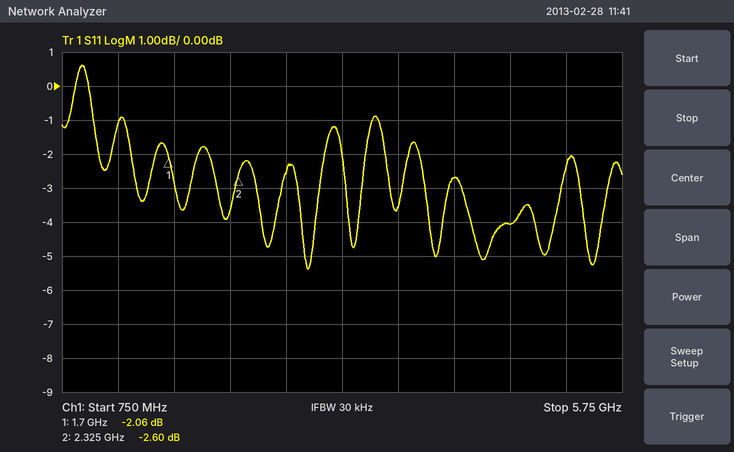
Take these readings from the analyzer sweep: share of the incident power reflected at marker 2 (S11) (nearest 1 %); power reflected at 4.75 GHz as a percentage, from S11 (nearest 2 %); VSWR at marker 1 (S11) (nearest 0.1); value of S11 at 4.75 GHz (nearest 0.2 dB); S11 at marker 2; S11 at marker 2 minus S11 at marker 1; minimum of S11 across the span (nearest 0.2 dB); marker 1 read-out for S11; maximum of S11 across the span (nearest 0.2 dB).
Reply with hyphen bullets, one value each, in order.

- 55 %
- 40 %
- 8.5
- -4.0 dB
- -2.60 dB
- -0.54 dB
- -5.4 dB
- -2.06 dB
- 0.6 dB
